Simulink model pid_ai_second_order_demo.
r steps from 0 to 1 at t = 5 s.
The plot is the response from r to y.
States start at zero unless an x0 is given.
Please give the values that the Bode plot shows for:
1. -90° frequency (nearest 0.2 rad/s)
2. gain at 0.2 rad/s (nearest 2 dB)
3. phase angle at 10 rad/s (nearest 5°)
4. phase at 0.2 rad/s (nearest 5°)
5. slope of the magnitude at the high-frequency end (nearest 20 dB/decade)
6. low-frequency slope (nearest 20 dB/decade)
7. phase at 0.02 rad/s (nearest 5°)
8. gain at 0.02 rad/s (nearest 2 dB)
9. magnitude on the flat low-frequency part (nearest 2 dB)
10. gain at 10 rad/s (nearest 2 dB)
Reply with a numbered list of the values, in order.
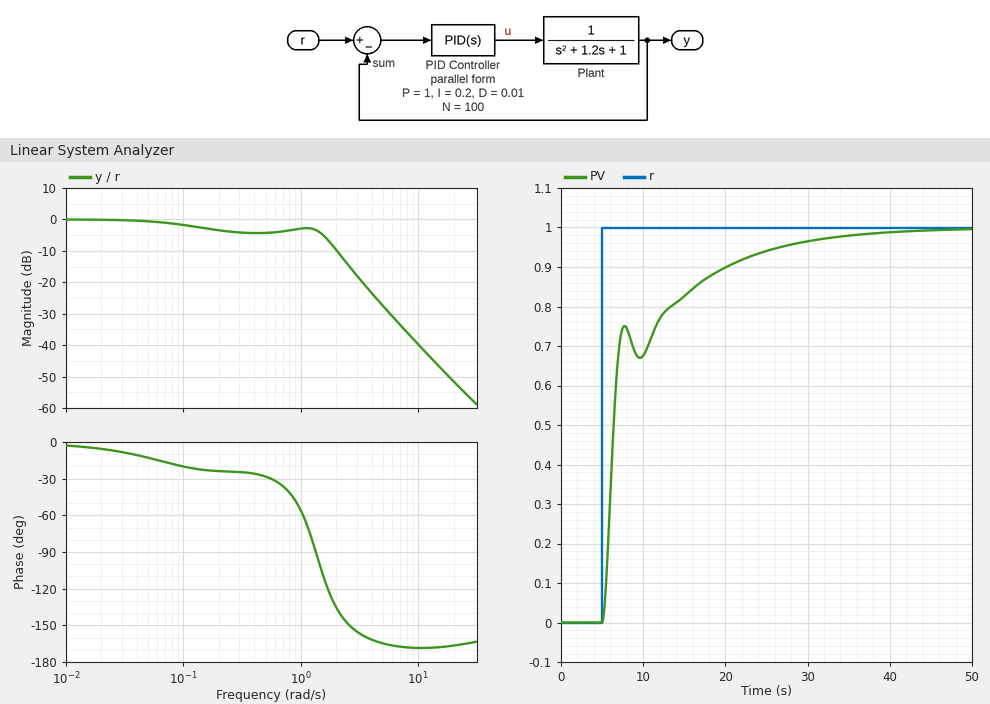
1. 1.4 rad/s
2. -4 dB
3. -170°
4. -25°
5. -40 dB/decade
6. 0 dB/decade
7. -5°
8. 0 dB
9. 0 dB
10. -40 dB
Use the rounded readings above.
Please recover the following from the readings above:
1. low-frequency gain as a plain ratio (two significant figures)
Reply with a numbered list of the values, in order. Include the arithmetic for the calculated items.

1. 10^(0 / 20) = 1.0
